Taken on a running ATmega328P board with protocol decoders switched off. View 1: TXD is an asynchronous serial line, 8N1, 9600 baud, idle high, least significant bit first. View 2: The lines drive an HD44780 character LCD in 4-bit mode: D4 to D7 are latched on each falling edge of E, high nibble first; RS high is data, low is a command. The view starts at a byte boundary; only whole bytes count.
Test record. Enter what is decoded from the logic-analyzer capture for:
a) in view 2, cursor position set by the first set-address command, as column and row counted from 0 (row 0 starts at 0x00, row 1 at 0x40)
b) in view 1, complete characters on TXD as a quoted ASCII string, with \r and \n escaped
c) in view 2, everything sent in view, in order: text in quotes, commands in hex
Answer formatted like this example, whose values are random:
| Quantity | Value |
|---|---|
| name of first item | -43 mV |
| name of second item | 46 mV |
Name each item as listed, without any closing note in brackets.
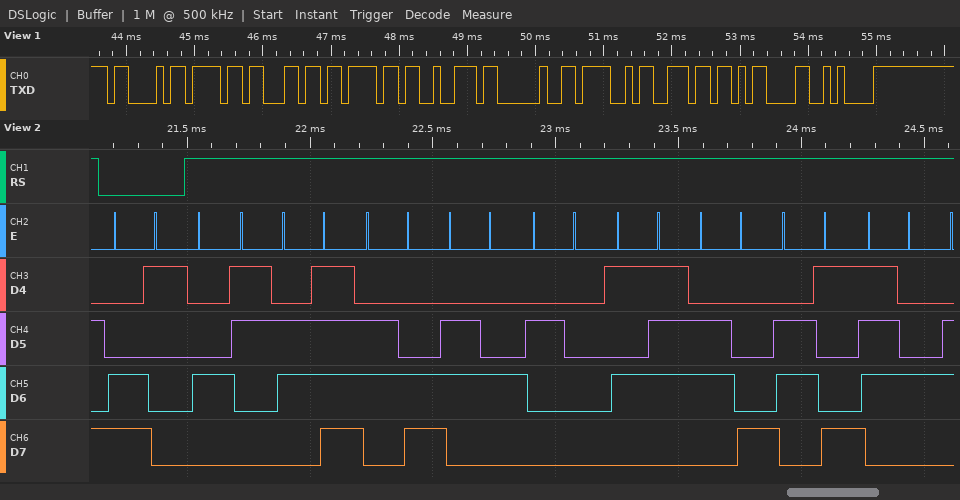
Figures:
| Quantity | Value |
|---|---|
| in view 2, cursor position set by the first set-address command, as column and row counted from 0 | column 1, row 1 |
| in view 1, complete characters on TXD as a quoted ASCII string, with \r and \n escaped | "Color On\r\n" |
| in view 2, everything sent in view, in order: text in quotes, commands in hex | 0xC1 "Cold Whit" |
